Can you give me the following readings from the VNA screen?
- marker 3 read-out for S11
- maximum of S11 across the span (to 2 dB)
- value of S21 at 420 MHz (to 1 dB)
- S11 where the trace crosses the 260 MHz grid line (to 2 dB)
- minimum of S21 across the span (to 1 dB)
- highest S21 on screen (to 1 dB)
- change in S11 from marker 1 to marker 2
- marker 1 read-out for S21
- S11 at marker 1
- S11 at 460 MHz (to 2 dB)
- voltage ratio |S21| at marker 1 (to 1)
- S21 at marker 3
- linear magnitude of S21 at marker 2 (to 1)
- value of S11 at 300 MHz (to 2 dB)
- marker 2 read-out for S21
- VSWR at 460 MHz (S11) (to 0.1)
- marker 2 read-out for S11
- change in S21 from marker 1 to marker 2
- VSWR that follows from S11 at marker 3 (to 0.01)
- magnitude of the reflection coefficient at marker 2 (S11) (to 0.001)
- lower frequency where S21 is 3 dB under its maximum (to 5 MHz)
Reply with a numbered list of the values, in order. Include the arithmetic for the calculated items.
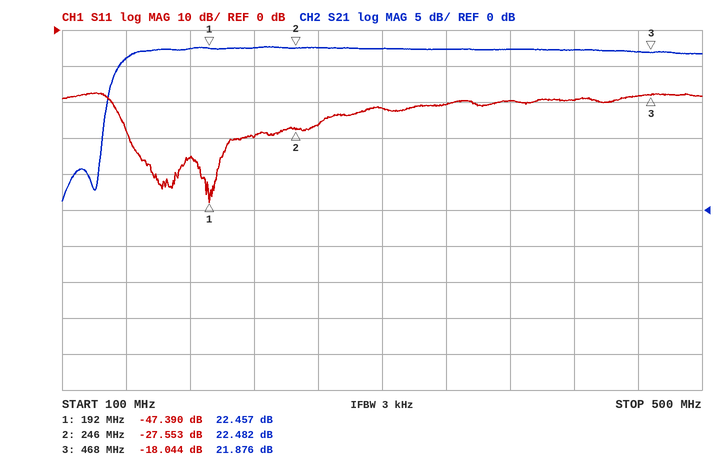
1. -18.044 dB
2. -18 dB
3. 22 dB
4. -26 dB
5. 1 dB
6. 23 dB
7. -27.553 − (-47.39) = 19.837 dB
8. 22.457 dB
9. -47.390 dB
10. -18 dB
11. 10^(22.457/20) ≈ 13
12. 21.876 dB
13. 10^(22.482/20) ≈ 13
14. -22 dB
15. 22.482 dB
16. |Γ| = 10^(-18/20) = 0.1259; VSWR = (1 + 0.1259)/(1 − 0.1259) ≈ 1.3
17. -27.553 dB
18. 22.482 − (22.457) = 0.025 dB
19. (1 + 0.1253)/(1 − 0.1253) ≈ 1.29
20. 10^(-27.553/20) ≈ 0.042
21. 135 MHz
